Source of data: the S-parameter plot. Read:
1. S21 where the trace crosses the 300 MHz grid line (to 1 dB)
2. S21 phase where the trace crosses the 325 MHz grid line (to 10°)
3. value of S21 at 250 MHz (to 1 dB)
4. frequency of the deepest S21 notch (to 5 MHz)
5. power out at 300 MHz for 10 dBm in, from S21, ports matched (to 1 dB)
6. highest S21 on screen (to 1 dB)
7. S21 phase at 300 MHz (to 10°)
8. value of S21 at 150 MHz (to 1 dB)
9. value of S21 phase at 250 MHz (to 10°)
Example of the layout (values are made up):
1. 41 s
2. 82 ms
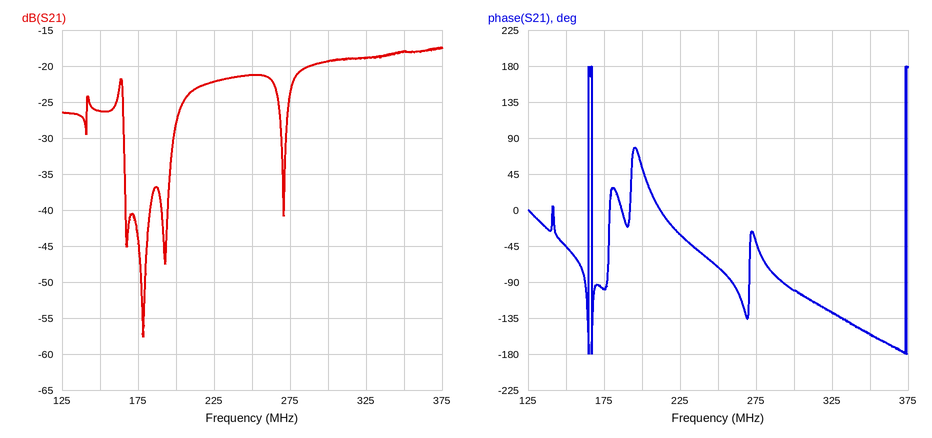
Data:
1. -19 dB
2. -130°
3. -21 dB
4. 180 MHz
5. -9 dBm
6. -17 dB
7. -100°
8. -26 dB
9. -70°
